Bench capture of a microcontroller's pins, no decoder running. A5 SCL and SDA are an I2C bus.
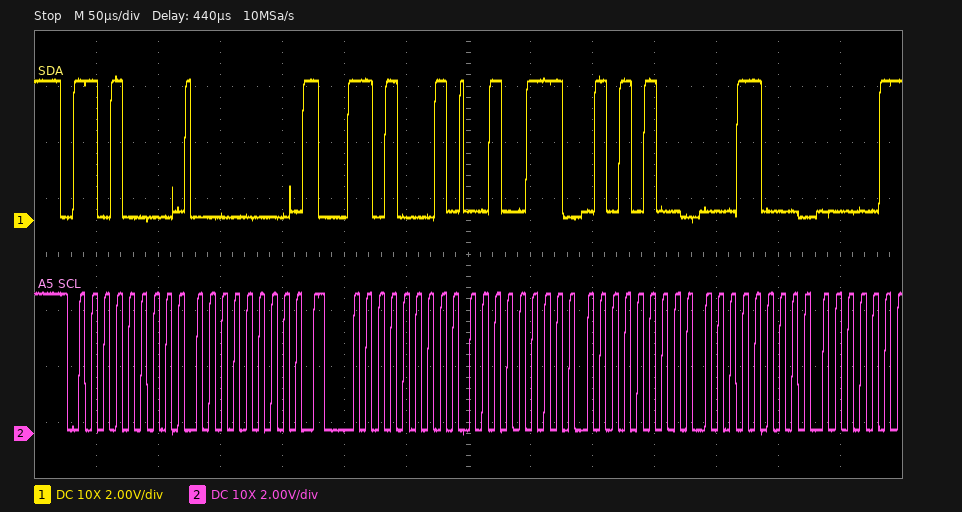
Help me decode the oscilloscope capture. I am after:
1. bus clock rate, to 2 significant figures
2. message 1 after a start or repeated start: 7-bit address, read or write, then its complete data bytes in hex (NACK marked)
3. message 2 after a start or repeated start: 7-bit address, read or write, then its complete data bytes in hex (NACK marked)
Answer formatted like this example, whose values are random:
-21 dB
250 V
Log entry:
100 kHz
0x68 write: 00
0x68 read: 27 54 18
